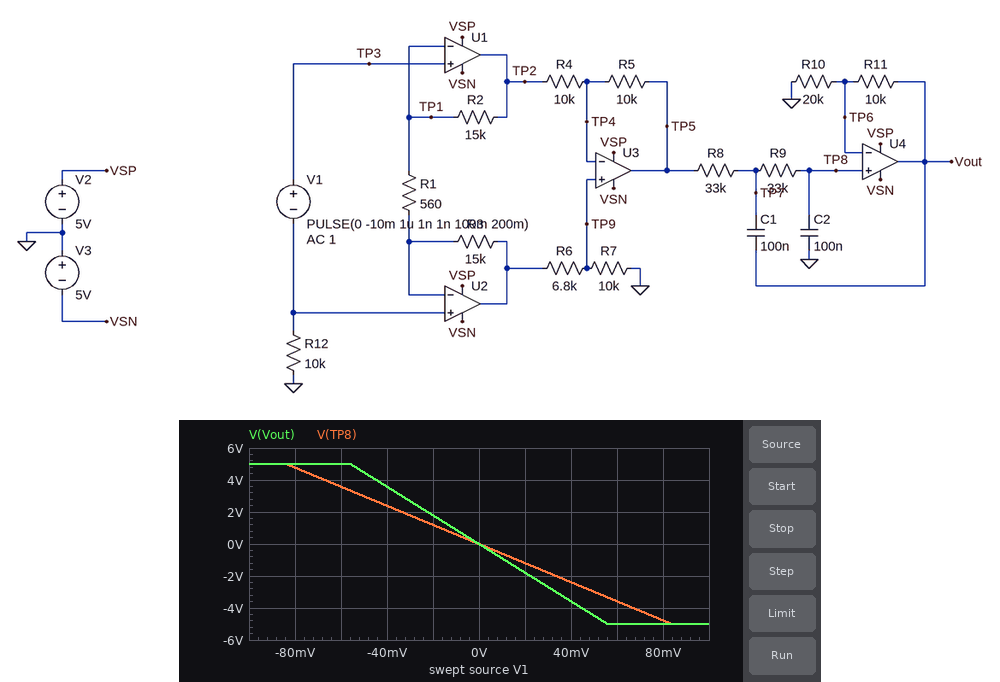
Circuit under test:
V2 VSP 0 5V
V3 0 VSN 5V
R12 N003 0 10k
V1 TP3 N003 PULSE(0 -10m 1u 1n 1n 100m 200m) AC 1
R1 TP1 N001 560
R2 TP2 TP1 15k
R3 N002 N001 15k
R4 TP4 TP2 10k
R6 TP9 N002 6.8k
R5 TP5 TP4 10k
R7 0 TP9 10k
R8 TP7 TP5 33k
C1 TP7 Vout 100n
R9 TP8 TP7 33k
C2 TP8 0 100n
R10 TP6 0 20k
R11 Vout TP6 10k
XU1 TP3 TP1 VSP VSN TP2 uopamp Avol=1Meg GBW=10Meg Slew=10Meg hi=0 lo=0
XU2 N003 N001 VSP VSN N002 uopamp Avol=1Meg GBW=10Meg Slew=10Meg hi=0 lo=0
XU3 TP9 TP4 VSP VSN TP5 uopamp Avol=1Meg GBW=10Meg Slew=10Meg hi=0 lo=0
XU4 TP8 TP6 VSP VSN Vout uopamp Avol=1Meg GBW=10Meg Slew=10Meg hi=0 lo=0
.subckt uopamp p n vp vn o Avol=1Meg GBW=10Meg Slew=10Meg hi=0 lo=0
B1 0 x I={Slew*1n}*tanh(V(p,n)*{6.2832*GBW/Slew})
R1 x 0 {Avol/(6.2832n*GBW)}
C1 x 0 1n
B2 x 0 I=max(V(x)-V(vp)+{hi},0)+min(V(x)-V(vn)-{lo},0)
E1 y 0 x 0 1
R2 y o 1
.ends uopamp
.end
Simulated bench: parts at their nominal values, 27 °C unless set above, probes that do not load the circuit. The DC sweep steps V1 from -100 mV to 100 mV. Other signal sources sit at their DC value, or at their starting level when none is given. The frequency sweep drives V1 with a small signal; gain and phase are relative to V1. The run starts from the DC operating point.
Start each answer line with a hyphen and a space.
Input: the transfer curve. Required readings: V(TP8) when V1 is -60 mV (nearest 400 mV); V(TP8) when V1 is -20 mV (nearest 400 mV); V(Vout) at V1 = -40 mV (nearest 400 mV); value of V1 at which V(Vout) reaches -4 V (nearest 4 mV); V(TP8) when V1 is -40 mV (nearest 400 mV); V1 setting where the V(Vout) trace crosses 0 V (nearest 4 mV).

- 3.6 V
- 1.2 V
- 3.6 V
- 44 mV
- 2.4 V
- 0 V
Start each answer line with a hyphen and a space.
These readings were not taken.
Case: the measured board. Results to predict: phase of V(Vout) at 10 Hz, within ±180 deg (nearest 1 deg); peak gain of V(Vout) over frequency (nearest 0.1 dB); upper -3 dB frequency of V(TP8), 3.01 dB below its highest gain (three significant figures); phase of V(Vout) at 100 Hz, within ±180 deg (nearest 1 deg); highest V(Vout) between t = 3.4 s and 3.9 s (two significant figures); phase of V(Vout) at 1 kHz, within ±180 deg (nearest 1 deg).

- 162 deg
- 39.0 dB
- 45.3 Hz
- 43 deg
- 920 mV
- 4 deg
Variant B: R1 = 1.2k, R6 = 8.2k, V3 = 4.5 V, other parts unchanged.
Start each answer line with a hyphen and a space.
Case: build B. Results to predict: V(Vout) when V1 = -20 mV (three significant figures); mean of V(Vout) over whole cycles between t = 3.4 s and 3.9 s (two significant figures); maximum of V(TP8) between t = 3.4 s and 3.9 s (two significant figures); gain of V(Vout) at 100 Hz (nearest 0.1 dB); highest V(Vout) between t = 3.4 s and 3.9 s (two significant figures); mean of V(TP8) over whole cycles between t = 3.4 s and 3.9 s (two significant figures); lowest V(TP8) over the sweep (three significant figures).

- 817 mV
- 200 mV
- 280 mV
- 19.1 dB
- 420 mV
- 140 mV
- -2.72 V
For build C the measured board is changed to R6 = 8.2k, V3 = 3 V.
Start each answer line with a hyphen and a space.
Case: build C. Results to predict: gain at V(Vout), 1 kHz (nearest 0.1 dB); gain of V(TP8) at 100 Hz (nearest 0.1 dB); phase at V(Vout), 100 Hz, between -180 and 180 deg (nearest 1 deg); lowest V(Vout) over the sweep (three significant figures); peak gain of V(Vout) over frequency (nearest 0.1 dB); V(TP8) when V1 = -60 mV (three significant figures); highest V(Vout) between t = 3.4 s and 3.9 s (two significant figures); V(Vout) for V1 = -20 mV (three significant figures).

- -14.0 dB
- 22.0 dB
- 43 deg
- -3.01 V
- 38.7 dB
- 3.43 V
- 880 mV
- 1.72 V
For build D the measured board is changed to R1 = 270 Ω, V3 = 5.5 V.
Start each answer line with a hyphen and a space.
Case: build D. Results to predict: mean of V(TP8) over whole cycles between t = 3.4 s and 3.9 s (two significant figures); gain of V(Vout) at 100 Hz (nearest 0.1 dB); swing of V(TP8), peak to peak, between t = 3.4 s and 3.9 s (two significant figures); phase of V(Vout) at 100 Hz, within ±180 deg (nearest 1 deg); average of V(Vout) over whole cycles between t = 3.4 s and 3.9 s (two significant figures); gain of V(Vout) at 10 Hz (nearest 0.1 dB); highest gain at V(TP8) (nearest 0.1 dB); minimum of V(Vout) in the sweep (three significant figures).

- 610 mV
- 32.2 dB
- 1.3 V
- 43 deg
- 920 mV
- 45.2 dB
- 41.8 dB
- -5.51 V
